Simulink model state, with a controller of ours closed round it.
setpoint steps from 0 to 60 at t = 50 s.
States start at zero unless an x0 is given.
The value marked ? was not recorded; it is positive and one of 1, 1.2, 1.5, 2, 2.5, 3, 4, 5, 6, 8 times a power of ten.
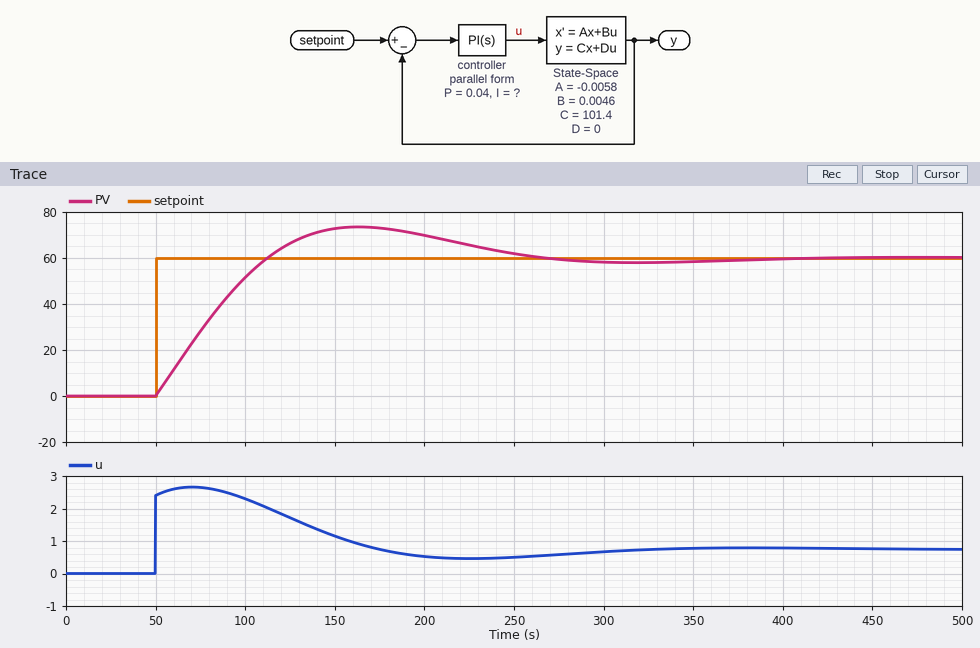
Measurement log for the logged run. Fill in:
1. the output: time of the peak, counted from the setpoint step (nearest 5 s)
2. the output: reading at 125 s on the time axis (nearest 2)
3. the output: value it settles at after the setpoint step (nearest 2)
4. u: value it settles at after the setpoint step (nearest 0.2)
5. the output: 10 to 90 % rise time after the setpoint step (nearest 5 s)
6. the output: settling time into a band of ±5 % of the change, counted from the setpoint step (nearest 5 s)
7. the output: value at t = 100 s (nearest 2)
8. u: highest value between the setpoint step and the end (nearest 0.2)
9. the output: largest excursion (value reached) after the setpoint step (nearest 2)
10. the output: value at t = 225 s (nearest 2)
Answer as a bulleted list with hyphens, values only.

- 115 s
- 66
- 60
- 0.8
- 50 s
- 190 s
- 52
- 2.6
- 74
- 66
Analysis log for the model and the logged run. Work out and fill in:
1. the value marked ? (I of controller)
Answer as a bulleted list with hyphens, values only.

- 0.0012
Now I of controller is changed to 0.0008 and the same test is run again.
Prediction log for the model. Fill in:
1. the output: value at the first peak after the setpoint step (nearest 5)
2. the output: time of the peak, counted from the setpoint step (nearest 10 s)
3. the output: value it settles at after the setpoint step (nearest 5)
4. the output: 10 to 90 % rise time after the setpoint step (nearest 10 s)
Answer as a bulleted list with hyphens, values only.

- 70
- 140 s
- 60
- 60 s
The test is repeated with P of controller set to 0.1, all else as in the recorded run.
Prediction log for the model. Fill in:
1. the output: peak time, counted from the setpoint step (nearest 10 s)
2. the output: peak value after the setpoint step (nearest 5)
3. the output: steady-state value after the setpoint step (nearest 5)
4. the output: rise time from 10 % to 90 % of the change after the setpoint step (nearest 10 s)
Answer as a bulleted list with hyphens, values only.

- 100 s
- 65
- 60
- 40 s
